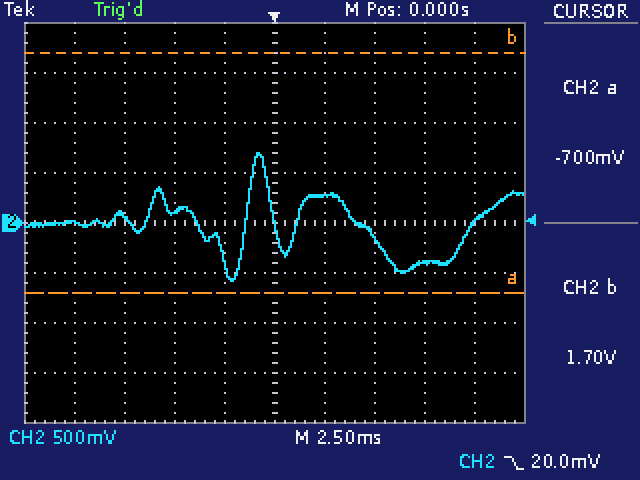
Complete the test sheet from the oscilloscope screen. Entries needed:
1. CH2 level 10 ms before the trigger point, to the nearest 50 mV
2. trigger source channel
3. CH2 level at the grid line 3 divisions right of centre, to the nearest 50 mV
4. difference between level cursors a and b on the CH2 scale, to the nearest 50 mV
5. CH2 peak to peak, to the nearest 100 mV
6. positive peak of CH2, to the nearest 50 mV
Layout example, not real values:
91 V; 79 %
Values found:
0 mV; CH2; -400 mV; 2.40 V; 1.30 V; 700 mV
